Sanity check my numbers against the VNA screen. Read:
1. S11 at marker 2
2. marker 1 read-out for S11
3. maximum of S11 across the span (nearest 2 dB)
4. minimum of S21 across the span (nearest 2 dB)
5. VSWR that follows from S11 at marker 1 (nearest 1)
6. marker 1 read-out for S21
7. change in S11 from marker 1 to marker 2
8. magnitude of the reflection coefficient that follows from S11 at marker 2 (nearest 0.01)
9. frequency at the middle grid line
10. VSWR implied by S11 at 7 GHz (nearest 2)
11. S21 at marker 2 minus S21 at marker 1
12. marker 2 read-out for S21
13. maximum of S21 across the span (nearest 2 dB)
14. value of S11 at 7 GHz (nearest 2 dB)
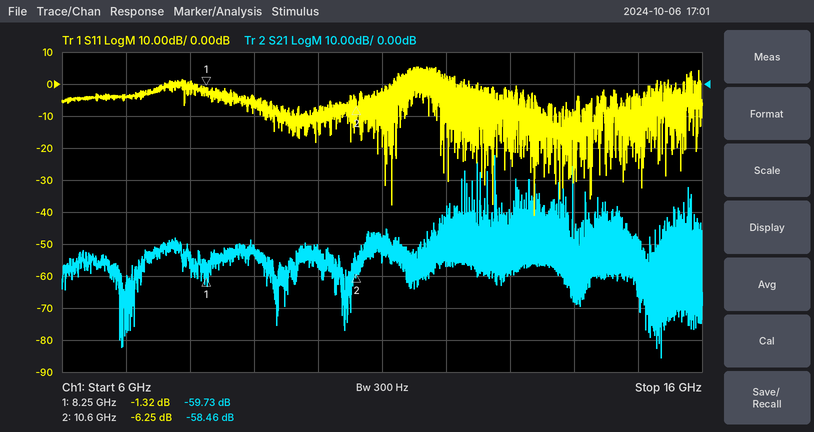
-6.25 dB
-1.32 dB
6 dB
-86 dB
13
-59.73 dB
-4.93 dB
0.49
11 GHz
4
1.27 dB
-58.46 dB
-22 dB
-4 dB
